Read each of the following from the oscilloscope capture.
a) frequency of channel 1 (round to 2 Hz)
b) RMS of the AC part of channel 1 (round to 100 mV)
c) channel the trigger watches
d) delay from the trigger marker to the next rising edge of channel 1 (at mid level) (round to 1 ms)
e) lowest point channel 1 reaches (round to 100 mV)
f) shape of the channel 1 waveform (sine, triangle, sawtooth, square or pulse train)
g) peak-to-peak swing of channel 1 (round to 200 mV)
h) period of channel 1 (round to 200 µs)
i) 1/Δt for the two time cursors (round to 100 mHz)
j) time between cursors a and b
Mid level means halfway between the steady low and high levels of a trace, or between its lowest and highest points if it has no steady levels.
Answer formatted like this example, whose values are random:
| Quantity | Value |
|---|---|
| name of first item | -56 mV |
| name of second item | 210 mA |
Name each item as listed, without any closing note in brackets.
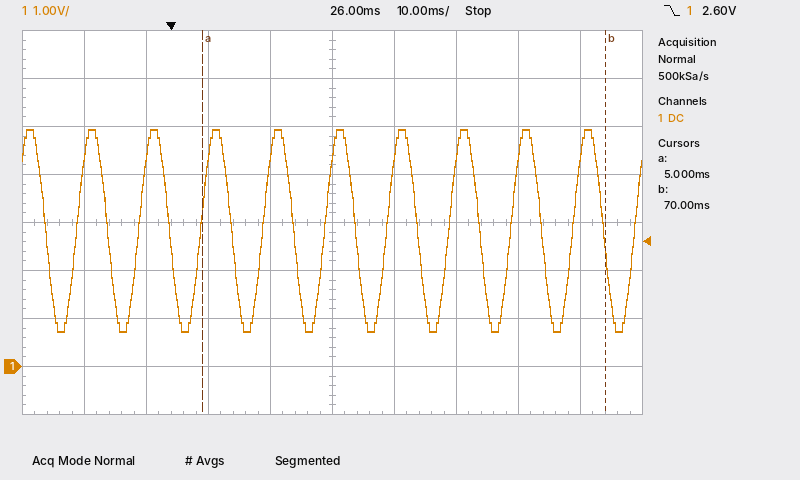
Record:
| Quantity | Value |
|---|---|
| frequency of channel 1 | 100 Hz |
| RMS of the AC part of channel 1 | 1.5 V |
| channel the trigger watches | channel 1 |
| delay from the trigger marker to the next rising edge of channel 1 (at mid level) | 5 ms |
| lowest point channel 1 reaches | 700 mV |
| shape of the channel 1 waveform | sine |
| peak-to-peak swing of channel 1 | 4.2 V |
| period of channel 1 | 10.0 ms |
| 1/Δt for the two time cursors | 15.4 Hz |
| time between cursors a and b | 65 ms |
